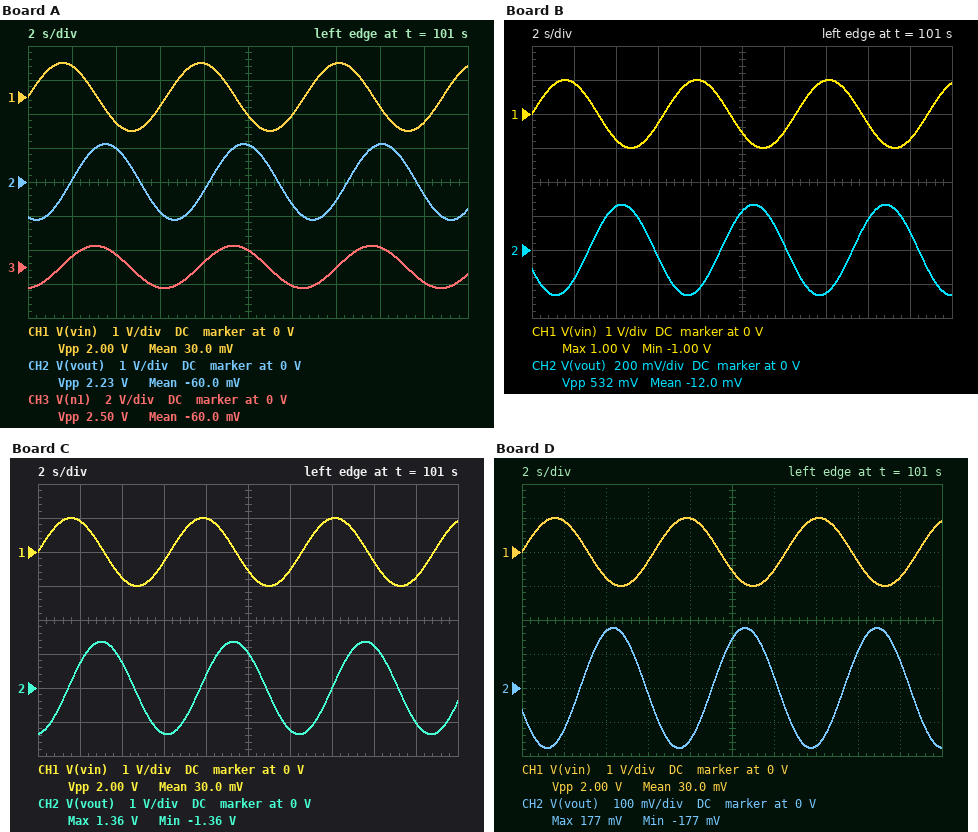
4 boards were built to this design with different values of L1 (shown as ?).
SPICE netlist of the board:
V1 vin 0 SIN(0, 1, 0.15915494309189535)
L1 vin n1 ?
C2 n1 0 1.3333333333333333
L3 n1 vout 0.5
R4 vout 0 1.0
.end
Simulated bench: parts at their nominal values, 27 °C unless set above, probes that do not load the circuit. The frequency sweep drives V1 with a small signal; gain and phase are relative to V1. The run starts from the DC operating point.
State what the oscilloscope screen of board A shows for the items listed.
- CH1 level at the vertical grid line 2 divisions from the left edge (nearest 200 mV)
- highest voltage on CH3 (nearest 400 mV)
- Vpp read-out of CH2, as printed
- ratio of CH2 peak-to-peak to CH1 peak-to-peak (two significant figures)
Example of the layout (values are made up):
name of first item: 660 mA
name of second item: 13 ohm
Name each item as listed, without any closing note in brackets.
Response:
CH1 level at the vertical grid line 2 divisions from the left edge: -800 mV
highest voltage on CH3: 1.2 V
Vpp read-out of CH2, as printed: 2.23 V
ratio of CH2 peak-to-peak to CH1 peak-to-peak: 1.1
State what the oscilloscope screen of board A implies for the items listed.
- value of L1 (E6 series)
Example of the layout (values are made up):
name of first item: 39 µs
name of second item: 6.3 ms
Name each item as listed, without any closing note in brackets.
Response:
value of L1: 1 H
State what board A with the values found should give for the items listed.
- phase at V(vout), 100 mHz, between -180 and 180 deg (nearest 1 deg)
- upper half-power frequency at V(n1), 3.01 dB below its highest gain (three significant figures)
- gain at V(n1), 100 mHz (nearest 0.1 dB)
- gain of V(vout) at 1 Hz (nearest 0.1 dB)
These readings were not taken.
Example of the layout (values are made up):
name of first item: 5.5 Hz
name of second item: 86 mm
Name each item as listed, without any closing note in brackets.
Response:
phase at V(vout), 100 mHz, between -180 and 180 deg: -59 deg
upper half-power frequency at V(n1), 3.01 dB below its highest gain: 206 mHz
gain at V(n1), 100 mHz: 1.2 dB
gain of V(vout) at 1 Hz: -44.3 dB
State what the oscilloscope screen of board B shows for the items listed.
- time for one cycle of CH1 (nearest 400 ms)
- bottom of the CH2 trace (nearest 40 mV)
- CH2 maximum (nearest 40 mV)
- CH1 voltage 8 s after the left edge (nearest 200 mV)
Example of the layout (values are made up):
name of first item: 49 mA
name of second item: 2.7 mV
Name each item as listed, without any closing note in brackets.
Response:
time for one cycle of CH1: 6.4 s
bottom of the CH2 trace: -280 mV
CH2 maximum: 280 mV
CH1 voltage 8 s after the left edge: 1.0 V
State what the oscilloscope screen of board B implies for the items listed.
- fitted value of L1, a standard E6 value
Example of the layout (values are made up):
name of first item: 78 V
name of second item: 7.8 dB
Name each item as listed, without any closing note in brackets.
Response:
fitted value of L1, a standard E6 value: 3.3 H
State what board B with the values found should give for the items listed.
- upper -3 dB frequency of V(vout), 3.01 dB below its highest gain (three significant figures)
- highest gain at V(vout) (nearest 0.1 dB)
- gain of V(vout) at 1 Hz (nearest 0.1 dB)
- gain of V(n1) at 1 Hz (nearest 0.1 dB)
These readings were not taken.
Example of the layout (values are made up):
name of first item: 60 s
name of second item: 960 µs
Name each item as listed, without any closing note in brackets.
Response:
upper -3 dB frequency of V(vout), 3.01 dB below its highest gain: 64.0 mHz
highest gain at V(vout): 0 dB
gain of V(vout) at 1 Hz: -54.8 dB
gain of V(n1) at 1 Hz: -44.4 dB
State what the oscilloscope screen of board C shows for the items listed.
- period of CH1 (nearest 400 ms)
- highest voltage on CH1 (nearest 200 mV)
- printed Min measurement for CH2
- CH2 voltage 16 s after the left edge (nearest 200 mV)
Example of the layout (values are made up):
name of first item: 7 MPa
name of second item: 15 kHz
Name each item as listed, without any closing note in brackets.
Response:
period of CH1: 6.4 s
highest voltage on CH1: 1.0 V
printed Min measurement for CH2: -1.36 V
CH2 voltage 16 s after the left edge: 1.2 V
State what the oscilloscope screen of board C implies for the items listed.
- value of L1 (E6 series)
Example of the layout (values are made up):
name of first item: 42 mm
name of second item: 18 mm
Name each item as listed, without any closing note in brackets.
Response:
value of L1: 680 mH
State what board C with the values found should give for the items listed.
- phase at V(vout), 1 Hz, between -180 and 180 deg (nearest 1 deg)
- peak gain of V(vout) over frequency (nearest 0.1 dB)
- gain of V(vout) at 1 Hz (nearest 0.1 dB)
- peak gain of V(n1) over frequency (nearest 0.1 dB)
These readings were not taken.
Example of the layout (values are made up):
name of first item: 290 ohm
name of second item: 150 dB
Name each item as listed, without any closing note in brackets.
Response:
phase at V(vout), 1 Hz, between -180 and 180 deg: 108 deg
peak gain of V(vout) over frequency: 3.1 dB
gain of V(vout) at 1 Hz: -40.9 dB
peak gain of V(n1) over frequency: 4.4 dB
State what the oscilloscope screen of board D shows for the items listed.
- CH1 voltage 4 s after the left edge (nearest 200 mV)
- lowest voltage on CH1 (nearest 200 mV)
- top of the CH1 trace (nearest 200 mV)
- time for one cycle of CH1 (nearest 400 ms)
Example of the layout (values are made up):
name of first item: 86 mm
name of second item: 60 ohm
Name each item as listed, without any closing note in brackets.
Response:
CH1 voltage 4 s after the left edge: -800 mV
lowest voltage on CH1: -1.0 V
top of the CH1 trace: 1.0 V
time for one cycle of CH1: 6.4 s
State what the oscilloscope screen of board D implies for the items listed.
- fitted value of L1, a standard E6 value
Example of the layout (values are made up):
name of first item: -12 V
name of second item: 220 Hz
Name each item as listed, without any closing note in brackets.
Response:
fitted value of L1, a standard E6 value: 4.7 H
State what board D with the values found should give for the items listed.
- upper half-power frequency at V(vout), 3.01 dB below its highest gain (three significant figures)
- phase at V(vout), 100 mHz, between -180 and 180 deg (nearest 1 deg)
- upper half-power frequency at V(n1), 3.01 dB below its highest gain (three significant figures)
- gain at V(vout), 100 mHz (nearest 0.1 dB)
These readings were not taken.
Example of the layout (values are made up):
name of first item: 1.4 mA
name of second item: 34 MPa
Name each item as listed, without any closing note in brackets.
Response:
upper half-power frequency at V(vout), 3.01 dB below its highest gain: 41.1 mHz
phase at V(vout), 100 mHz, between -180 and 180 deg: -121 deg
upper half-power frequency at V(n1), 3.01 dB below its highest gain: 41.8 mHz
gain at V(vout), 100 mHz: -9.2 dB
